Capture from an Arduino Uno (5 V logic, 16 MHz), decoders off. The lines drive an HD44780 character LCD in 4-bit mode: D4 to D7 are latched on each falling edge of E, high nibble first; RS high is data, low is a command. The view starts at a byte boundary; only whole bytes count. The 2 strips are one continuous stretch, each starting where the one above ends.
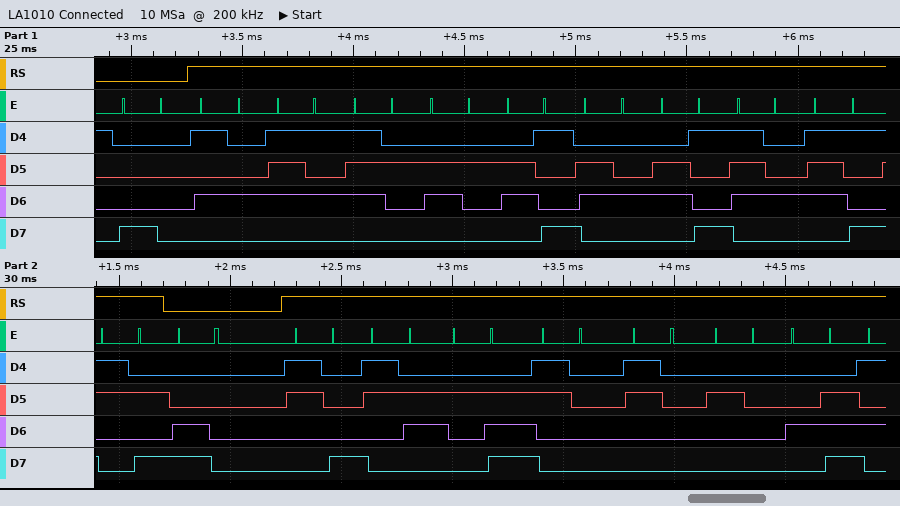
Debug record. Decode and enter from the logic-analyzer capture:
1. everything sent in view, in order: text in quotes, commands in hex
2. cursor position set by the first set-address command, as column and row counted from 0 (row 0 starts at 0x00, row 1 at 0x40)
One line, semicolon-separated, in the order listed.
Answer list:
0x80 "Turbidity:" 0xC0 "86.00 N"; column 0, row 0
